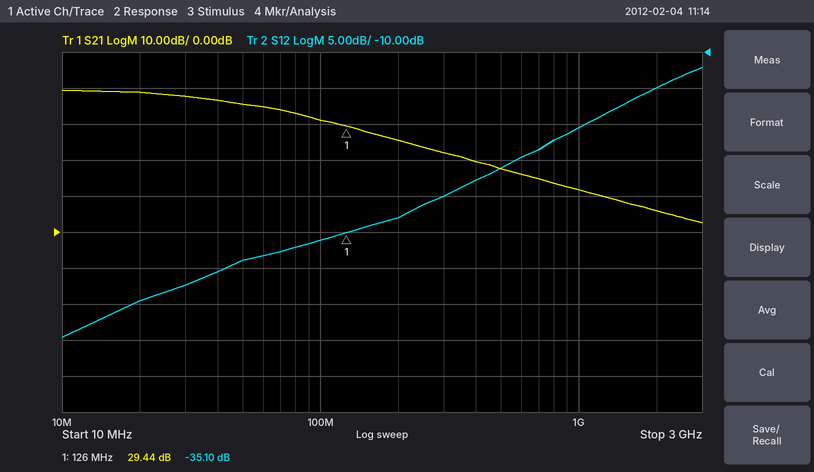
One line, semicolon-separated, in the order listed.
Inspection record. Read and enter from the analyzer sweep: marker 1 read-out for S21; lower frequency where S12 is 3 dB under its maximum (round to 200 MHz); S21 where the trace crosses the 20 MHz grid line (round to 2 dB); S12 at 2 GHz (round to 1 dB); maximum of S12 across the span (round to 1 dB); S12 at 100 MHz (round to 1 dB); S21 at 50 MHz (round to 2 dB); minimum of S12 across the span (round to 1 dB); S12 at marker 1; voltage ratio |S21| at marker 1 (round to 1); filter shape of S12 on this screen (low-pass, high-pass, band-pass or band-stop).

29.44 dB; 2.0 GHz; 38 dB; -15 dB; -12 dB; -36 dB; 36 dB; -50 dB; -35.10 dB; 30; high-pass
